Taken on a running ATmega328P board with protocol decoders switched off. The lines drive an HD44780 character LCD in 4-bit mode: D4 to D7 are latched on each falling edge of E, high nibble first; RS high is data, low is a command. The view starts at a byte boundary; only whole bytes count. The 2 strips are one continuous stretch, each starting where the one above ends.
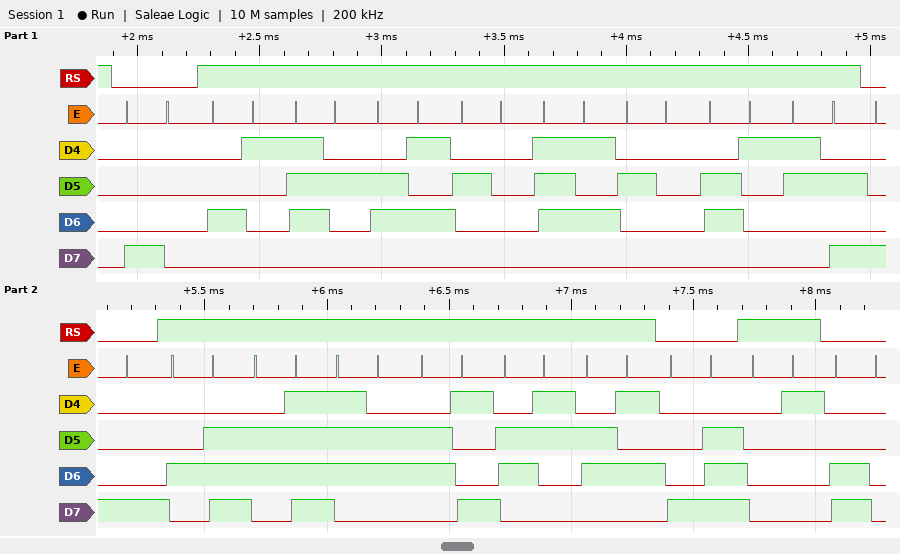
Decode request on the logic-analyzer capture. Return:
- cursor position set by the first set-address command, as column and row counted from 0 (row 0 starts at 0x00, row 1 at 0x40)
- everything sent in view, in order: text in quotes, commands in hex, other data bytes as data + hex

column 0, row 0
0x80 "Are u a:" 0x88 "Novice" 0x8E data 01 0xC0
